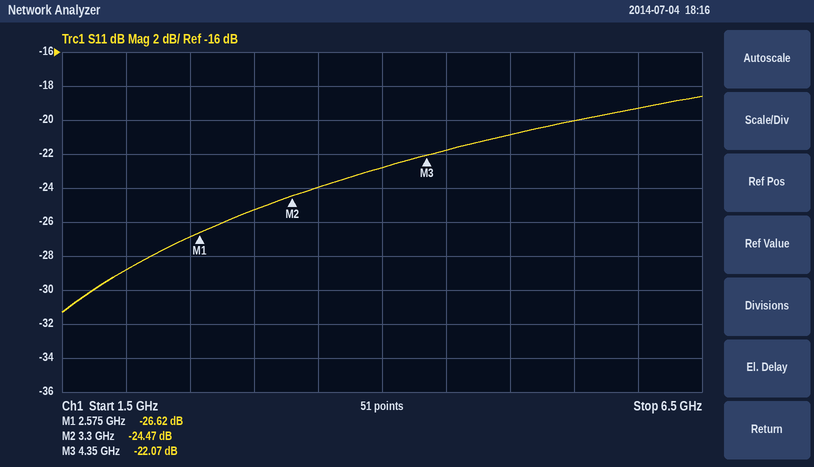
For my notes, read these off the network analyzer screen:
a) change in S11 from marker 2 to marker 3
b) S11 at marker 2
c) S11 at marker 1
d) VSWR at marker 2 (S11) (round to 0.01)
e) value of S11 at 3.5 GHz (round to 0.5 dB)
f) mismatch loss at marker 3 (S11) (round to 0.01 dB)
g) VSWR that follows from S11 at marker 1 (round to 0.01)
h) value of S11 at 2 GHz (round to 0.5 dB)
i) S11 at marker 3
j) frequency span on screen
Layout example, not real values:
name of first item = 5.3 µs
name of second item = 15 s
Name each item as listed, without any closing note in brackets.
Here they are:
change in S11 from marker 2 to marker 3 = 2.40 dB
S11 at marker 2 = -24.47 dB
S11 at marker 1 = -26.62 dB
VSWR at marker 2 (S11) = 1.13
value of S11 at 3.5 GHz = -24.0 dB
mismatch loss at marker 3 (S11) = 0.03 dB
VSWR that follows from S11 at marker 1 = 1.10
value of S11 at 2 GHz = -29.0 dB
S11 at marker 3 = -22.07 dB
frequency span on screen = 5 GHz
